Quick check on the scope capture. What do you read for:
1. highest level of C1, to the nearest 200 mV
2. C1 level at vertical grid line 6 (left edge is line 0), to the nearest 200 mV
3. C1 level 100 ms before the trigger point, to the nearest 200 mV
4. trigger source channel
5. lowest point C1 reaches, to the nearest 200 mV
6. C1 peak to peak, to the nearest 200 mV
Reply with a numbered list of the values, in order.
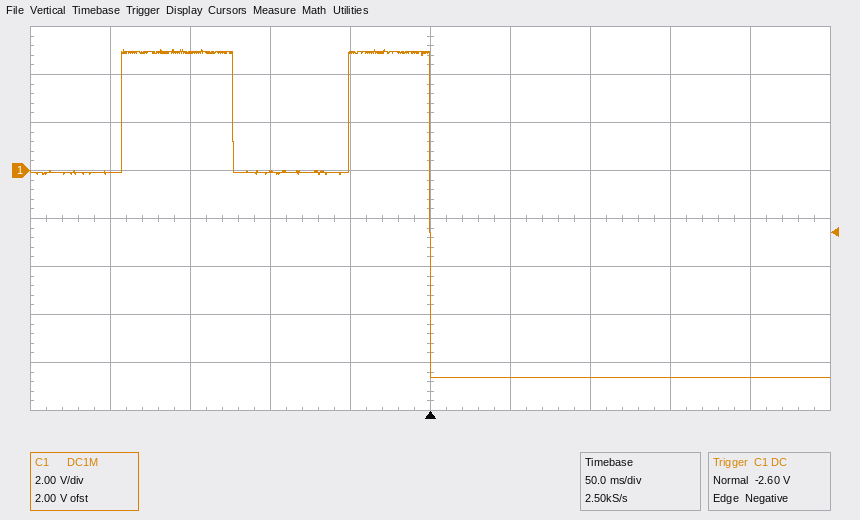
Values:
1. 5.0 V
2. -8.6 V
3. 0.0 V
4. C1
5. -8.6 V
6. 13.6 V
